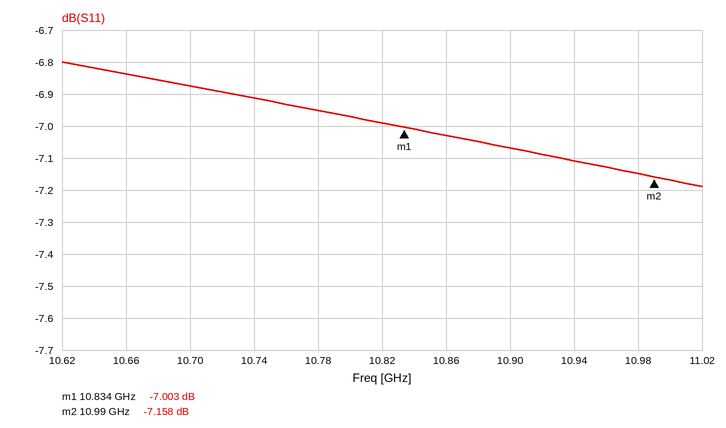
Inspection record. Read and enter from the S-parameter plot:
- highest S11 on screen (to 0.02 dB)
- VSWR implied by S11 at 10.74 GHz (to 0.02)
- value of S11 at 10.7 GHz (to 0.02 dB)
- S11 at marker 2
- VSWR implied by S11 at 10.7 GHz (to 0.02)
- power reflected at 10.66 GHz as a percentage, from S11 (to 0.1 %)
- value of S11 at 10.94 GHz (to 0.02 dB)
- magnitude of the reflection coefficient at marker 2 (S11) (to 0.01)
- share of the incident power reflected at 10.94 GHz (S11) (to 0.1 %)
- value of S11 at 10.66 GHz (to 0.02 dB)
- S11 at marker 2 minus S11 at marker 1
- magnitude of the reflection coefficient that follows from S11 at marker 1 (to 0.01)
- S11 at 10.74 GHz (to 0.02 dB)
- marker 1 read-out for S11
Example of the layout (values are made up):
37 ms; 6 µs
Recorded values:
-6.80 dB; 2.64; -6.88 dB; -7.158 dB; 2.66; 20.7 %; -7.10 dB; 0.44; 19.5 %; -6.84 dB; -0.155 dB; 0.45; -6.92 dB; -7.003 dB
